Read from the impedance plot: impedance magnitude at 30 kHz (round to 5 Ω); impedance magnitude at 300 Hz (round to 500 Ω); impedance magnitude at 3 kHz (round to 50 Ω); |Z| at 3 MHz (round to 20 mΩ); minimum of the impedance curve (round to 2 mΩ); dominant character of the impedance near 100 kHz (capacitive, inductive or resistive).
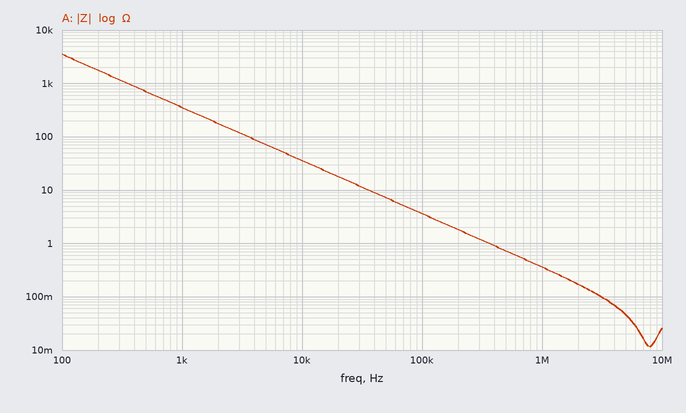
10 Ω
1.0 kΩ
100 Ω
100 mΩ
12 mΩ
capacitive
